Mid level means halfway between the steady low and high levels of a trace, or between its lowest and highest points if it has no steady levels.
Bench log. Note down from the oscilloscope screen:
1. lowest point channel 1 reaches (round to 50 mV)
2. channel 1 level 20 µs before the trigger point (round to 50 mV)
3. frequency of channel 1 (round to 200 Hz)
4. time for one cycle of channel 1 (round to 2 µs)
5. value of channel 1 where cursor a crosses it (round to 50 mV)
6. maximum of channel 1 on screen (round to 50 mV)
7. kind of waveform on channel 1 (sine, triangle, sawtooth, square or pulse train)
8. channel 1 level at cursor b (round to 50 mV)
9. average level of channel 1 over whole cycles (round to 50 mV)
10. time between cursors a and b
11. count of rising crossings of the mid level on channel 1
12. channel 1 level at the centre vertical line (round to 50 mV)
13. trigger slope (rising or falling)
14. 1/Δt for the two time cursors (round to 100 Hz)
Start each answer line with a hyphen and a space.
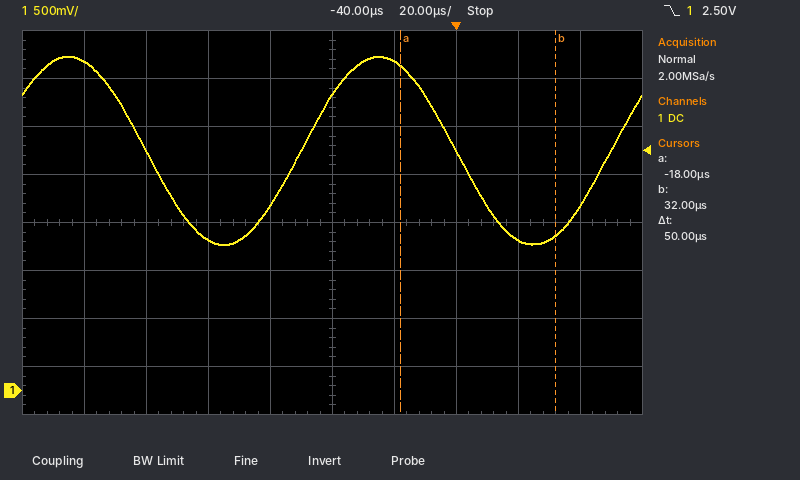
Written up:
- 1.50 V
- 3.45 V
- 10.0 kHz
- 100 µs
- 3.40 V
- 3.50 V
- sine
- 1.60 V
- 2.50 V
- 50 µs
- 2
- 3.10 V
- falling
- 20.0 kHz
